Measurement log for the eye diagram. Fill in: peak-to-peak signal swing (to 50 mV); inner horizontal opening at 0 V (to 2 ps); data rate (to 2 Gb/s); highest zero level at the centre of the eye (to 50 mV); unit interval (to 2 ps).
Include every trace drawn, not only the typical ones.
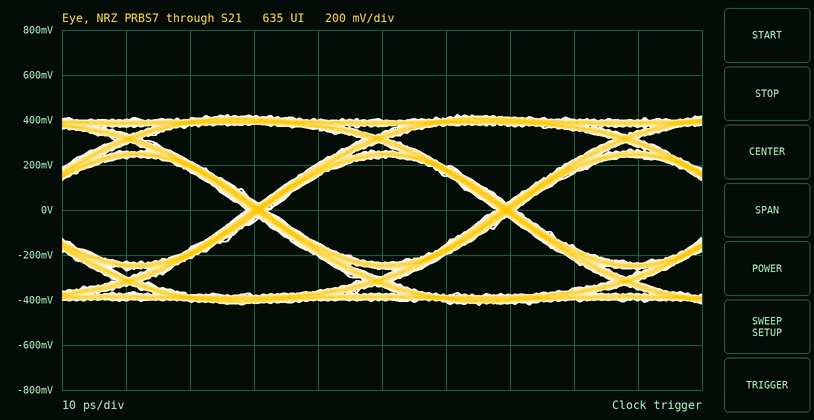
850 mV
36 ps
26 Gb/s
-250 mV
38 ps
